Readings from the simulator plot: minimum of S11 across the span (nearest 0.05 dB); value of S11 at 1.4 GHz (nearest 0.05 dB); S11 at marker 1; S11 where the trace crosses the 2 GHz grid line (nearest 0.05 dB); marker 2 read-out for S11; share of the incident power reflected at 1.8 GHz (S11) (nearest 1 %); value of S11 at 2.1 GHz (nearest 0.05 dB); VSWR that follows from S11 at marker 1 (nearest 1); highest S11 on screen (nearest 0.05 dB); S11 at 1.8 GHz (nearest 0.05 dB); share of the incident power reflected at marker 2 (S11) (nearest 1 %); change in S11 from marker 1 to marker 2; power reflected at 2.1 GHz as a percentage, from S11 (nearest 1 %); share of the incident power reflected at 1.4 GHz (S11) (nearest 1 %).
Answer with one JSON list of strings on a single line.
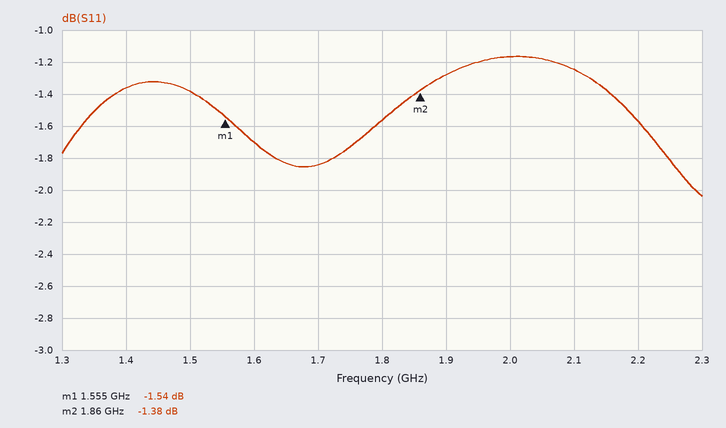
["-2.05 dB", "-1.35 dB", "-1.54 dB", "-1.15 dB", "-1.38 dB", "70 %", "-1.25 dB", "11", "-1.15 dB", "-1.55 dB", "73 %", "0.16 dB", "75 %", "73 %"]
